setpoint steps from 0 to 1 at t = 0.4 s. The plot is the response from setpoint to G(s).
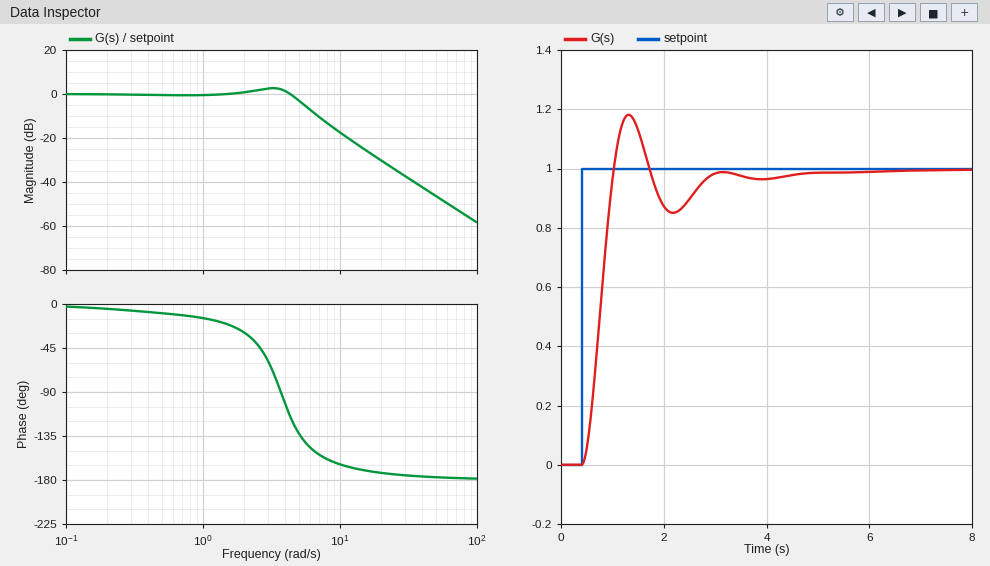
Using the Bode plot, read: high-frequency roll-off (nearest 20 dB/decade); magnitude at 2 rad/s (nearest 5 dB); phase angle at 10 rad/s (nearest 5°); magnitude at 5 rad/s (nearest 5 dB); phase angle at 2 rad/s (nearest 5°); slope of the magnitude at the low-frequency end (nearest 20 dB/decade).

-40 dB/decade
0 dB
-165°
-5 dB
-30°
0 dB/decade
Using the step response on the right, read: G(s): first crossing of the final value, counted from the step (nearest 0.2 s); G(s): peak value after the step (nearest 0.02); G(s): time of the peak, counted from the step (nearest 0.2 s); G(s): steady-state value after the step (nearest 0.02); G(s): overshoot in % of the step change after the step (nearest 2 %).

0.6 s
1.18
1.0 s
1.00
18 %
